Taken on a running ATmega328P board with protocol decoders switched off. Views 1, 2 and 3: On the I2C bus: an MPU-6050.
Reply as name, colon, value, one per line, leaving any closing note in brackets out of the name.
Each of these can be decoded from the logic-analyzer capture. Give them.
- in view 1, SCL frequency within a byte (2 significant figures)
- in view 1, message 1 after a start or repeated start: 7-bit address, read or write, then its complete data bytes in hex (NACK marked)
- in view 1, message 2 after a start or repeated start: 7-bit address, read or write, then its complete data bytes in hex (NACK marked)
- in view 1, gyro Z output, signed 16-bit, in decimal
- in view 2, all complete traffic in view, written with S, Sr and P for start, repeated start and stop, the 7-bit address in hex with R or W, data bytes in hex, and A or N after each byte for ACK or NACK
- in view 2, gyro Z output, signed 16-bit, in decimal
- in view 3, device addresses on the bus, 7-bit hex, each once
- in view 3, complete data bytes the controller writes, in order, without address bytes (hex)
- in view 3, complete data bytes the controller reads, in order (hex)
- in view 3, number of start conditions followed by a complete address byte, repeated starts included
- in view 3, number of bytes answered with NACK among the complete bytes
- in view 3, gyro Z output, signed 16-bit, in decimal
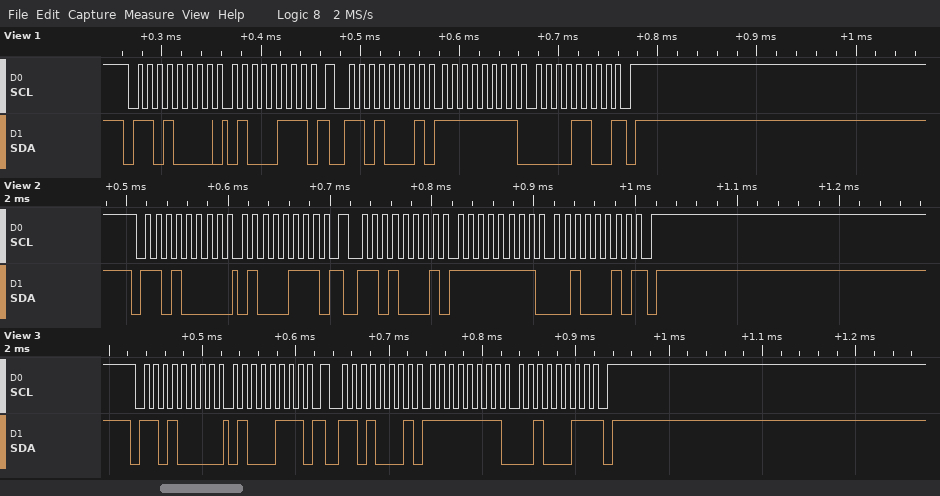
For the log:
in view 1, SCL frequency within a byte: 100 kHz
in view 1, message 1 after a start or repeated start: 7-bit address, read or write, then its complete data bytes in hex: 0x68 write: 47
in view 1, message 2 after a start or repeated start: 7-bit address, read or write, then its complete data bytes in hex: 0x68 read: FF 0C NACK
in view 1, gyro Z output, signed 16-bit, in decimal: -244
in view 2, all complete traffic in view, written with S, Sr and P for start, repeated start and stop, the 7-bit address in hex with R or W, data bytes in hex, and A or N after each byte for ACK or NACK: S 68W A 47 A Sr 68R A FF A 22 N P
in view 2, gyro Z output, signed 16-bit, in decimal: -222
in view 3, device addresses on the bus, 7-bit hex, each once: 0x68
in view 3, complete data bytes the controller writes, in order, without address bytes: 47
in view 3, complete data bytes the controller reads, in order: FF 23
in view 3, number of start conditions followed by a complete address byte, repeated starts included: 2
in view 3, number of bytes answered with NACK among the complete bytes: 1
in view 3, gyro Z output, signed 16-bit, in decimal: -221
